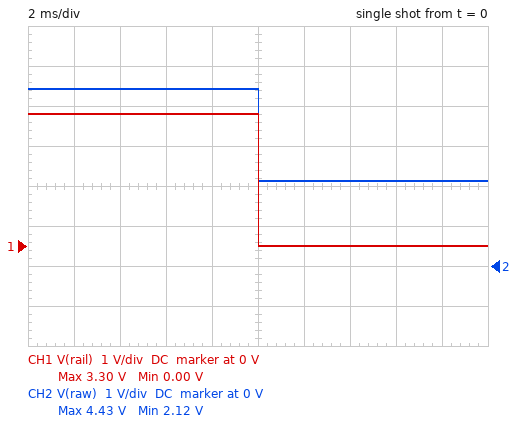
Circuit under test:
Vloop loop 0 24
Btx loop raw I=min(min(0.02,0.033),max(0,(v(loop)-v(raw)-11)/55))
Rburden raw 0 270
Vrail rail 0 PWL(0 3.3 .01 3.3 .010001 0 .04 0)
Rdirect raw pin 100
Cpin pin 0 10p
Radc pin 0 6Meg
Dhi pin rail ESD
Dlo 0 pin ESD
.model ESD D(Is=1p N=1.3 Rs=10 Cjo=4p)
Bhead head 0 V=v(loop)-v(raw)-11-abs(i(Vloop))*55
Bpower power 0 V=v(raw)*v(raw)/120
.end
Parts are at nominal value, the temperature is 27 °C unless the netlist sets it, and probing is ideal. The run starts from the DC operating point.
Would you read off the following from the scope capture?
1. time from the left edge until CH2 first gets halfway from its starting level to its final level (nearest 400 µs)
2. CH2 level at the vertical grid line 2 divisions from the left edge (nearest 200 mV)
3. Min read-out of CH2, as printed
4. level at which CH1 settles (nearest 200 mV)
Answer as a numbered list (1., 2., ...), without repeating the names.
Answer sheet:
1. 10.0 ms
2. 4.4 V
3. 2.12 V
4. 0 V
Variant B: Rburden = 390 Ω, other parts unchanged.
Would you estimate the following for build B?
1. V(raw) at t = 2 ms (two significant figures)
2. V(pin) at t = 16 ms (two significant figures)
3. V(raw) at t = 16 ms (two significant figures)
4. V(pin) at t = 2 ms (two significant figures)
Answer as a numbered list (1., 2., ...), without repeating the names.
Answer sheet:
1. 4.9 V
2. 930 mV
3. 2.3 V
4. 4.1 V
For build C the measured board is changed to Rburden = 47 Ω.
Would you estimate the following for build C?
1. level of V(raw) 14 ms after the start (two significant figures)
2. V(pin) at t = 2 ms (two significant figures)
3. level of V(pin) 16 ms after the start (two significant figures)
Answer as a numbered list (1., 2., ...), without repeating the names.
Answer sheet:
1. 870 mV
2. 940 mV
3. 720 mV
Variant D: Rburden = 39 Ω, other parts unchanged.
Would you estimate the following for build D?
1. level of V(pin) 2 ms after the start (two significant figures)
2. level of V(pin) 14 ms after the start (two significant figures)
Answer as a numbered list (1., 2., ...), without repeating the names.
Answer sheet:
1. 780 mV
2. 690 mV
